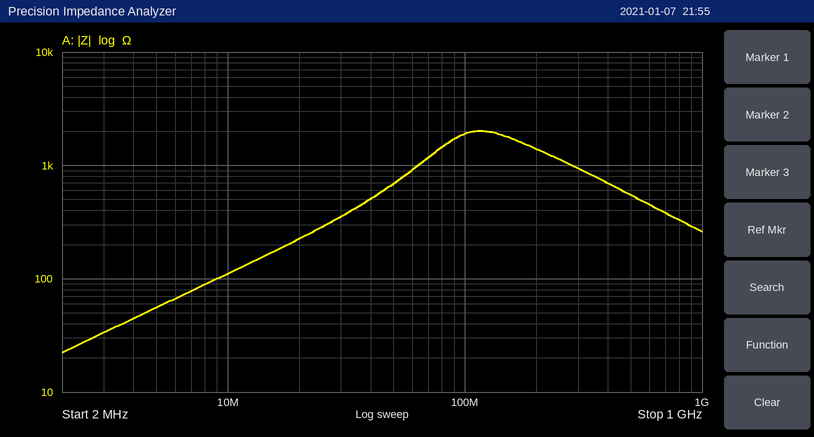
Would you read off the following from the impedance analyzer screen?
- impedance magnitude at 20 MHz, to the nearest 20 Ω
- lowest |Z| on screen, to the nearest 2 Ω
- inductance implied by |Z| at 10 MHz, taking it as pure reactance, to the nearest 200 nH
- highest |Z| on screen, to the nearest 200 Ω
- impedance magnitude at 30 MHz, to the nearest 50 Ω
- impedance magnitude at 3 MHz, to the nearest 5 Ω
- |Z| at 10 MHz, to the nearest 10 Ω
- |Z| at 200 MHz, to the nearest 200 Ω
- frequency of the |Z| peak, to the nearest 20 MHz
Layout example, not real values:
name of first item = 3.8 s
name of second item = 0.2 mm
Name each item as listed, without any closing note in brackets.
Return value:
impedance magnitude at 20 MHz, to the nearest 20 Ω = 220 Ω
lowest |Z| on screen, to the nearest 2 Ω = 22 Ω
inductance implied by |Z| at 10 MHz, taking it as pure reactance, to the nearest 200 nH = 1.8 µH
highest |Z| on screen, to the nearest 200 Ω = 2.0 kΩ
impedance magnitude at 30 MHz, to the nearest 50 Ω = 350 Ω
impedance magnitude at 3 MHz, to the nearest 5 Ω = 35 Ω
|Z| at 10 MHz, to the nearest 10 Ω = 110 Ω
|Z| at 200 MHz, to the nearest 200 Ω = 1.4 kΩ
frequency of the |Z| peak, to the nearest 20 MHz = 120 MHz
